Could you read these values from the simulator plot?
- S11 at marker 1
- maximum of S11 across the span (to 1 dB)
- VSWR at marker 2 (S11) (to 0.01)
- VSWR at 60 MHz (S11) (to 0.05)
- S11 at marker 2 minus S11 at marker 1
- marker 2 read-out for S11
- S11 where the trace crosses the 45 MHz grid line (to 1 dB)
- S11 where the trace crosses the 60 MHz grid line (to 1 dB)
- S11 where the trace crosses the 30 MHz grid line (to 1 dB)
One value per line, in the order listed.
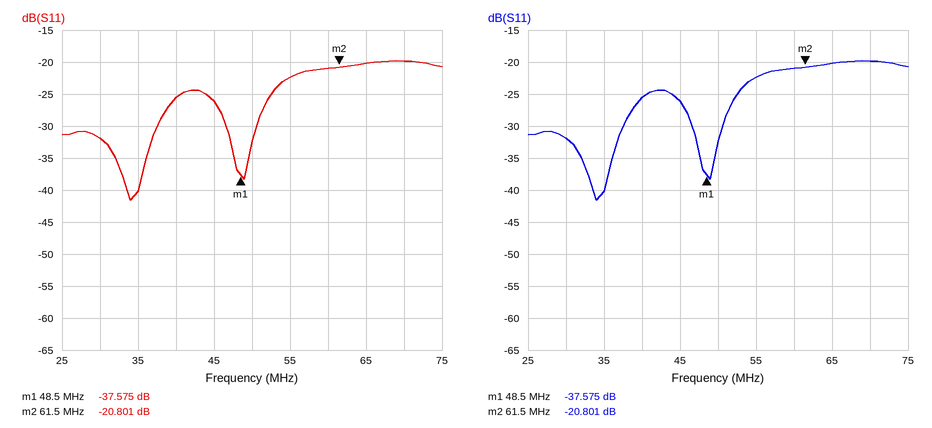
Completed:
-37.575 dB
-20 dB
1.20
1.20
16.774 dB
-20.801 dB
-26 dB
-21 dB
-32 dB
